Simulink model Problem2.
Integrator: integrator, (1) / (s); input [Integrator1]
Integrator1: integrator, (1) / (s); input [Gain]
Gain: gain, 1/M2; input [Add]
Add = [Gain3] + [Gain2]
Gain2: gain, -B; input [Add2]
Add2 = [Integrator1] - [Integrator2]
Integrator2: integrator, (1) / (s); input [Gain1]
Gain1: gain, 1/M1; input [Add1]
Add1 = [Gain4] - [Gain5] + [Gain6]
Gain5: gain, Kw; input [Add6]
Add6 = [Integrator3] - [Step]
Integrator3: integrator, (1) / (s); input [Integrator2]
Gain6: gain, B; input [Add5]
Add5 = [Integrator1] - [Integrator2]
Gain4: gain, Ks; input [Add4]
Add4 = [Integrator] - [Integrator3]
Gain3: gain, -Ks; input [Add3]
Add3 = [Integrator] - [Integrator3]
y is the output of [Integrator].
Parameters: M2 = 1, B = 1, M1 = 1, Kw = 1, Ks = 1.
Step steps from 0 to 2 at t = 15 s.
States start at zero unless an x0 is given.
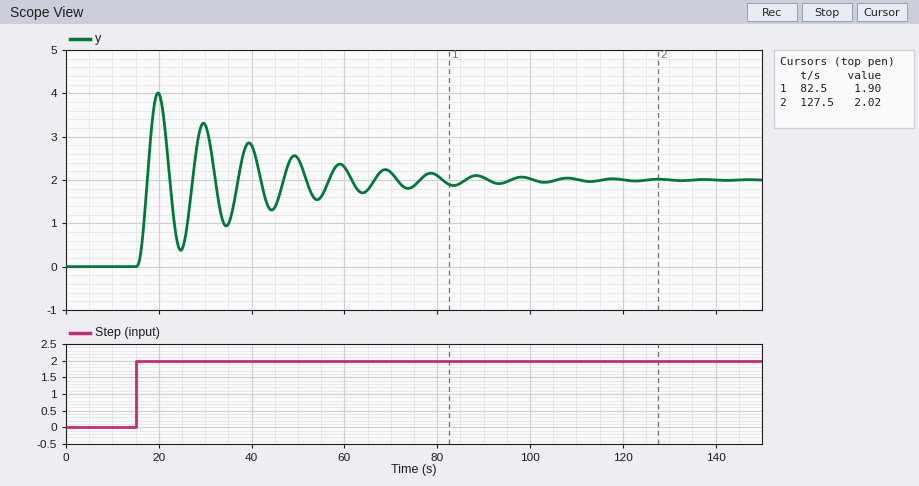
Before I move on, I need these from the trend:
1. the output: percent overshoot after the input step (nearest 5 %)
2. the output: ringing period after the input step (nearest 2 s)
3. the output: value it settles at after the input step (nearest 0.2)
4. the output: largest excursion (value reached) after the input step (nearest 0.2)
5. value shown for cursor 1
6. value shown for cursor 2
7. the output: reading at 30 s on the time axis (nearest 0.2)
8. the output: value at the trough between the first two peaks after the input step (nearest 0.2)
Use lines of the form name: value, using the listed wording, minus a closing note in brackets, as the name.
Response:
the output: percent overshoot after the input step: 100 %
the output: ringing period after the input step: 10 s
the output: value it settles at after the input step: 2.0
the output: largest excursion (value reached) after the input step: 4.0
value shown for cursor 1: 1.90
value shown for cursor 2: 2.02
the output: reading at 30 s on the time axis: 3.2
the output: value at the trough between the first two peaks after the input step: 0.4
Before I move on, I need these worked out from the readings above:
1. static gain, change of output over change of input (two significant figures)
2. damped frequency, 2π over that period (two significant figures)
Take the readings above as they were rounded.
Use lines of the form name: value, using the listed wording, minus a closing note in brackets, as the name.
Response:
static gain, change of output over change of input: 1.0
damped frequency, 2π over that period: 0.63 rad/s
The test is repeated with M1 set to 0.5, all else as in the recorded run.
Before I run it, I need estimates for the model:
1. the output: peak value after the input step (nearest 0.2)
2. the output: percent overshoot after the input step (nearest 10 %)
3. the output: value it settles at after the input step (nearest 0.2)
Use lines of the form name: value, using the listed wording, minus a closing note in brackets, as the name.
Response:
the output: peak value after the input step: 3.8
the output: percent overshoot after the input step: 90 %
the output: value it settles at after the input step: 2.0
